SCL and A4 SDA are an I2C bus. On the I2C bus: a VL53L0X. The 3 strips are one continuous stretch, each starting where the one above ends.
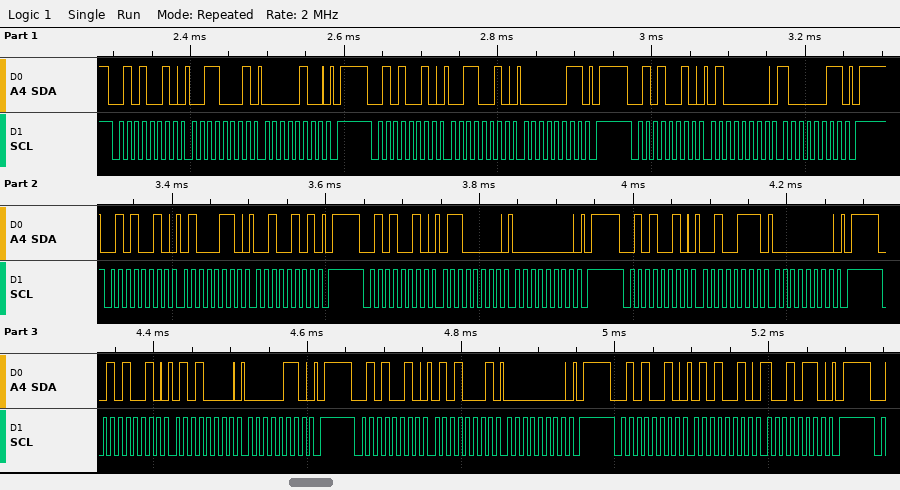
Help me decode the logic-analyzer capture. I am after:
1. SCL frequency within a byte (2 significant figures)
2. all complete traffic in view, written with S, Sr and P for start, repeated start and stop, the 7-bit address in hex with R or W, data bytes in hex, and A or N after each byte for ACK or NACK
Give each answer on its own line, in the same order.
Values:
100 kHz
S 29W A 31 A 04 A P S 29W A 32 A 03 A P S 29W A 40 A 83 A P S 29W A 46 A 25 A P S 29W A 60 A 00 A P S 29W A 27 A 00 A P S 29W A 50 A 06 A P S 29W A 51 A 00 A P S 29W A 52 A 96 A P
